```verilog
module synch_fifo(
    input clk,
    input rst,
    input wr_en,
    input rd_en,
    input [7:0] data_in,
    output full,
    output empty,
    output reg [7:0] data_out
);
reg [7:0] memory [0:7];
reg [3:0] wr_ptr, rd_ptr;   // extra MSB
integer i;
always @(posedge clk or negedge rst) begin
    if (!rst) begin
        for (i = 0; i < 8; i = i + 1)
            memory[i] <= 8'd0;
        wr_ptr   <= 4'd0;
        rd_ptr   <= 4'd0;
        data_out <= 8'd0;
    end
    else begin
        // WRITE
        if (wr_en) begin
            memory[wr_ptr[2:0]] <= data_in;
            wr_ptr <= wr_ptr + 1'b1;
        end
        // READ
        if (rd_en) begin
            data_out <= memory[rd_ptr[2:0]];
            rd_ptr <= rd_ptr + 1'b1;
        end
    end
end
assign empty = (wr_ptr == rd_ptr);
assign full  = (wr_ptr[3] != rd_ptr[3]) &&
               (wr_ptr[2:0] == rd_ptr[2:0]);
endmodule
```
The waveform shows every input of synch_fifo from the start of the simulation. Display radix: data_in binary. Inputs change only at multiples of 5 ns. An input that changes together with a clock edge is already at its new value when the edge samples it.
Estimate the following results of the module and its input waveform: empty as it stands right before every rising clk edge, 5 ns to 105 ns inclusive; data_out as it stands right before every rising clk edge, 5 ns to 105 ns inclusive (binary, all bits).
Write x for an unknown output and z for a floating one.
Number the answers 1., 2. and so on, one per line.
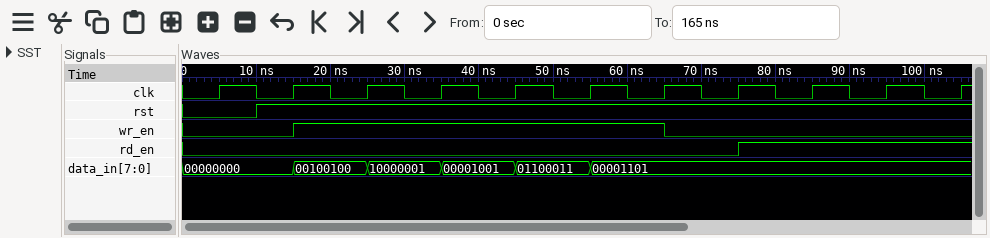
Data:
1. 1 1 0 0 0 0 0 0 0 0 0
2. 00000000, 00000000, 00000000, 00000000, 00000000, 00000000, 00000000, 00000000, 00100100, 10000001, 00001001
